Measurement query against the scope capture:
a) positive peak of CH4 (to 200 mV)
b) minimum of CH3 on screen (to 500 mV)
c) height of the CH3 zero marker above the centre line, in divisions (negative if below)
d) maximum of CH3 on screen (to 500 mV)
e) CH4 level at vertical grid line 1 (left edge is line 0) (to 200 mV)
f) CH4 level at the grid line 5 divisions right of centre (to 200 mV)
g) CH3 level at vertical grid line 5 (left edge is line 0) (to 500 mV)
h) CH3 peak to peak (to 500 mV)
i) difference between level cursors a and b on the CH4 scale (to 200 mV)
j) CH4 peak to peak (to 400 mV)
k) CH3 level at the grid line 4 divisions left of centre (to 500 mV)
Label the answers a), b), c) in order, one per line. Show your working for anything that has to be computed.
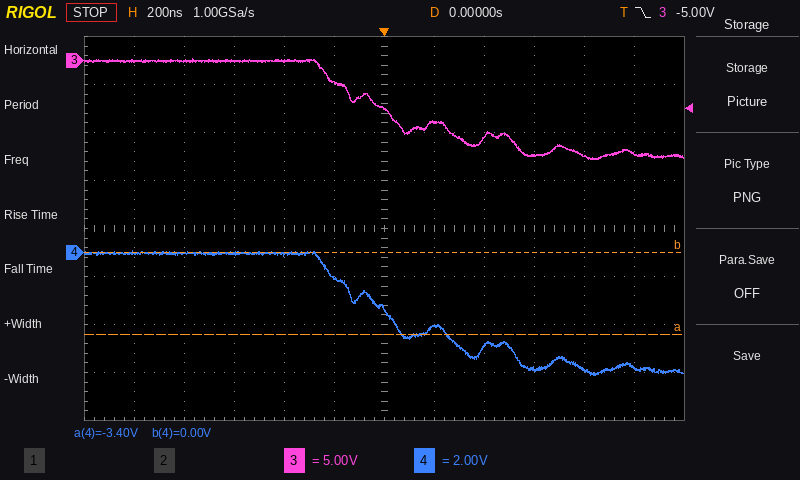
a) 0.0 V
b) -10.5 V
c) +3.5 div
d) 0.0 V
e) 0.0 V
f) -4.8 V
g) -2.5 V
h) 0.0 V − (-10.5 V) = 10.5 V
i) 3.4 V
j) 5.2 V
k) 0.0 V
